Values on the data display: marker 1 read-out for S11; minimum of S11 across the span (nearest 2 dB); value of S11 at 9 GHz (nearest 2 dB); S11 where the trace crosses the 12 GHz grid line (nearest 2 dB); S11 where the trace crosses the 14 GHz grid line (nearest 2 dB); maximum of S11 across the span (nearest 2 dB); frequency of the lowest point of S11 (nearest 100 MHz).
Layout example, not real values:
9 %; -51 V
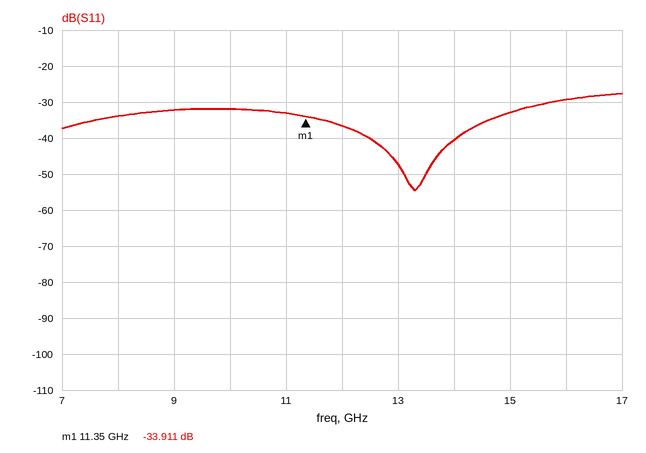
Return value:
-33.911 dB; -54 dB; -32 dB; -36 dB; -40 dB; -28 dB; 13.3 GHz
